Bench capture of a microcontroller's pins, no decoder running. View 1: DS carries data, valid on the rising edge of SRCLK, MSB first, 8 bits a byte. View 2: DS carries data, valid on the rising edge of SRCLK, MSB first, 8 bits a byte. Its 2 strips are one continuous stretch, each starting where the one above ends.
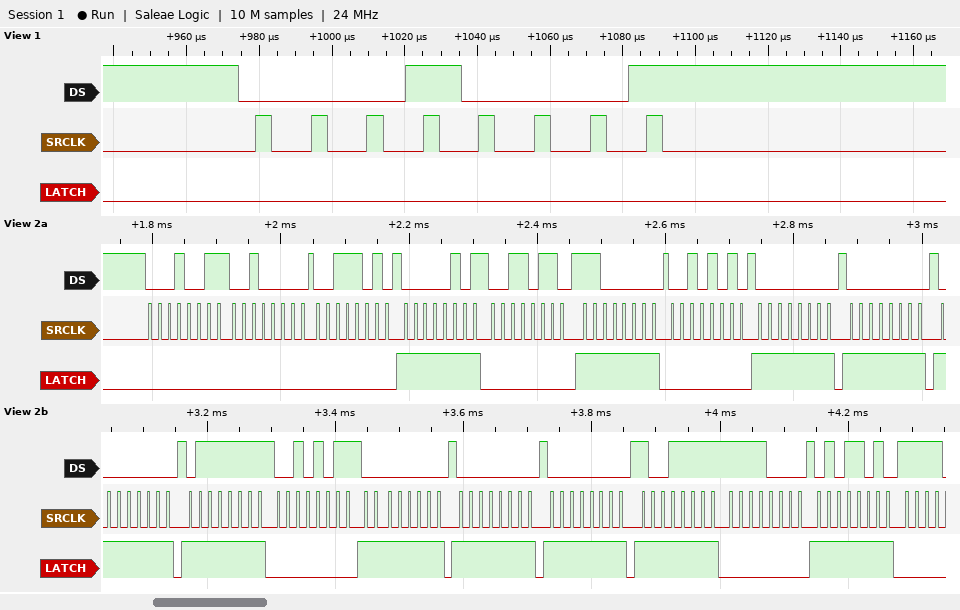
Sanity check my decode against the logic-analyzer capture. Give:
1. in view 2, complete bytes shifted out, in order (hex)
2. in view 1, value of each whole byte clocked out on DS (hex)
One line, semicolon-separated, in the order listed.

0x13 0x20 0x3A 0x05 0x36 0xC0 0x2A 0x00 0x00 0x00 0x7F 0x2B 0x00 0x00 0x00 0x9F 0xF0 0x5A; 11
